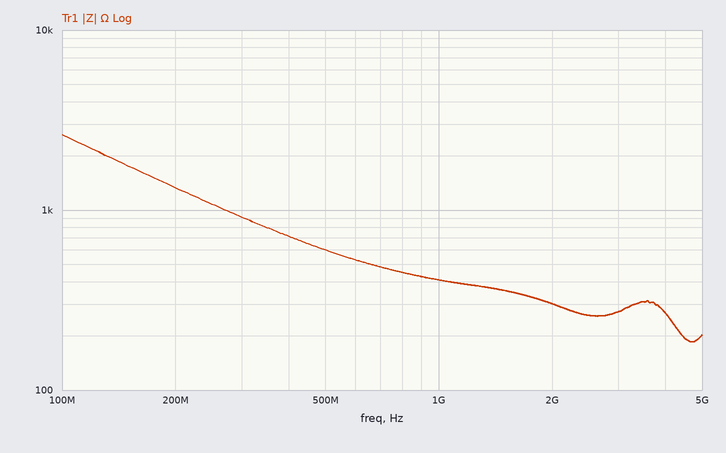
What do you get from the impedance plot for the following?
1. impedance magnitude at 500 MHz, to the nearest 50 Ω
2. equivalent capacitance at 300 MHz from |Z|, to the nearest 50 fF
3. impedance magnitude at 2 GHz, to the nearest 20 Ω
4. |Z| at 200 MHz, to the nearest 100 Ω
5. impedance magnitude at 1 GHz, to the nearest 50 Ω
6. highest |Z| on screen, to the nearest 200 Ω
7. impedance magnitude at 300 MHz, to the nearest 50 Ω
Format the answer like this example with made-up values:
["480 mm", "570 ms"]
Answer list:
["600 Ω", "600 fF", "300 Ω", "1.3 kΩ", "400 Ω", "2.6 kΩ", "900 Ω"]
